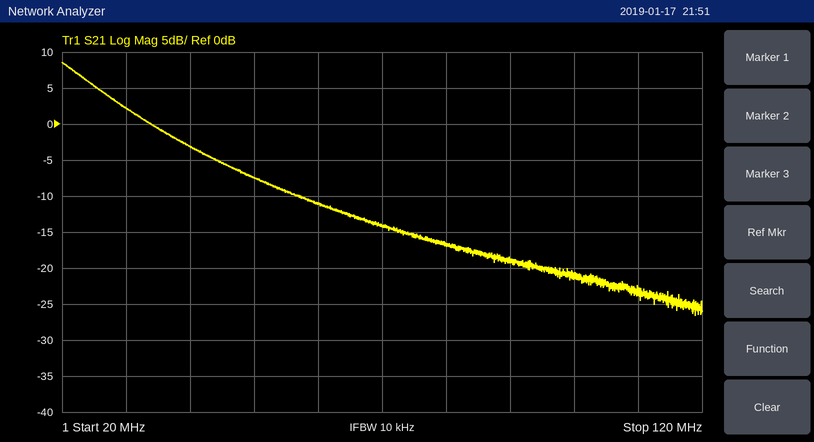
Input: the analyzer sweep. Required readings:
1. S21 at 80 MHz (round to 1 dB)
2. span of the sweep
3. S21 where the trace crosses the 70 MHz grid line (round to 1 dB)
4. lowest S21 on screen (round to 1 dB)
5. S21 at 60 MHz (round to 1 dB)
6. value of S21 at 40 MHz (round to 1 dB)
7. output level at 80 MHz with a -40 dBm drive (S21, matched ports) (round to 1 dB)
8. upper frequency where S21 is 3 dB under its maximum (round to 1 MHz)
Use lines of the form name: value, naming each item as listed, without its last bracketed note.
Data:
S21 at 80 MHz: -17 dB
span of the sweep: 100 MHz
S21 where the trace crosses the 70 MHz grid line: -14 dB
lowest S21 on screen: -27 dB
S21 at 60 MHz: -11 dB
value of S21 at 40 MHz: -3 dB
output level at 80 MHz with a -40 dBm drive (S21, matched ports): -57 dBm
upper frequency where S21 is 3 dB under its maximum: 25 MHz
